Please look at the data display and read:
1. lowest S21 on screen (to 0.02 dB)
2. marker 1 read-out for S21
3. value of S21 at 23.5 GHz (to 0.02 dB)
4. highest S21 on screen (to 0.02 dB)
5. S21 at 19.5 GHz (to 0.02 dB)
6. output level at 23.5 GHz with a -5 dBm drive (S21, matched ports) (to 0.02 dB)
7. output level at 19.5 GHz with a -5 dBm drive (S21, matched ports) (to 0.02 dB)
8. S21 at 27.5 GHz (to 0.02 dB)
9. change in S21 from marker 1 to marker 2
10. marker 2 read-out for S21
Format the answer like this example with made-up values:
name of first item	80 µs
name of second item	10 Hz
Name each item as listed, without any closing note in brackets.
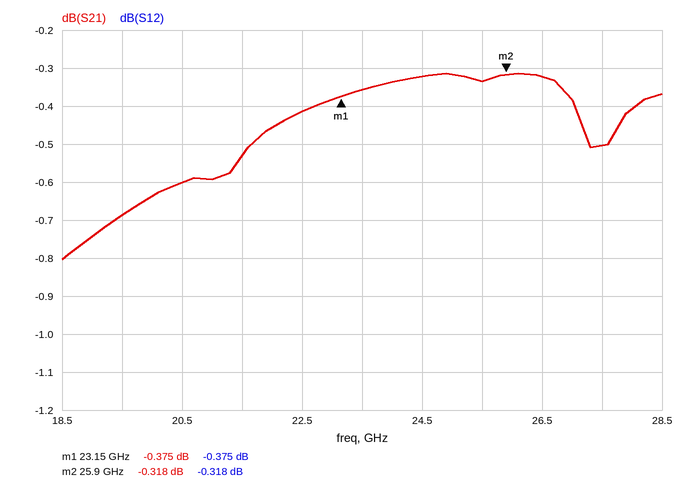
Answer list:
lowest S21 on screen	-0.80 dB
marker 1 read-out for S21	-0.375 dB
value of S21 at 23.5 GHz	-0.36 dB
highest S21 on screen	-0.32 dB
S21 at 19.5 GHz	-0.68 dB
output level at 23.5 GHz with a -5 dBm drive (S21, matched ports)	-5.36 dBm
output level at 19.5 GHz with a -5 dBm drive (S21, matched ports)	-5.68 dBm
S21 at 27.5 GHz	-0.50 dB
change in S21 from marker 1 to marker 2	0.057 dB
marker 2 read-out for S21	-0.318 dB
